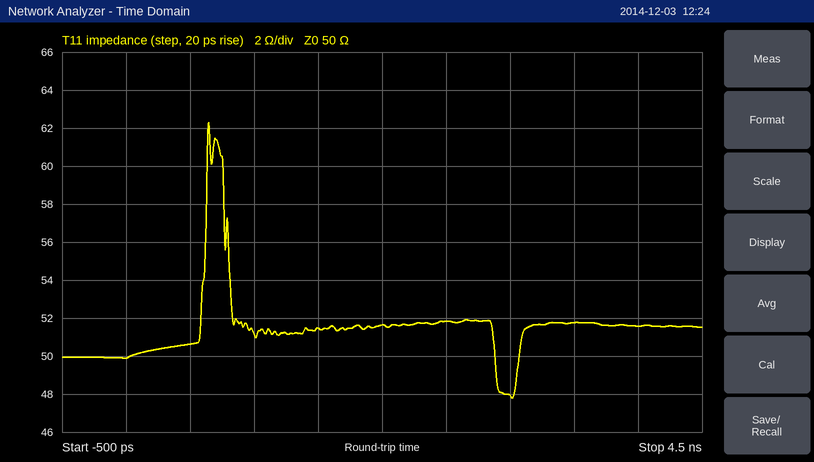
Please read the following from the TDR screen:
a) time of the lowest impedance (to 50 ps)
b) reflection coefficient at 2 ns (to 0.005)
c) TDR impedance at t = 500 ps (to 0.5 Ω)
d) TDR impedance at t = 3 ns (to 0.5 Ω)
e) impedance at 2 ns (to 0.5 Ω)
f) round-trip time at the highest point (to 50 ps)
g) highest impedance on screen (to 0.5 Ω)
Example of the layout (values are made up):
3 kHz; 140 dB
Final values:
3.00 ns; +0.015; 50.5 Ω; 48.0 Ω; 51.5 Ω; 650 ps; 62.5 Ω
